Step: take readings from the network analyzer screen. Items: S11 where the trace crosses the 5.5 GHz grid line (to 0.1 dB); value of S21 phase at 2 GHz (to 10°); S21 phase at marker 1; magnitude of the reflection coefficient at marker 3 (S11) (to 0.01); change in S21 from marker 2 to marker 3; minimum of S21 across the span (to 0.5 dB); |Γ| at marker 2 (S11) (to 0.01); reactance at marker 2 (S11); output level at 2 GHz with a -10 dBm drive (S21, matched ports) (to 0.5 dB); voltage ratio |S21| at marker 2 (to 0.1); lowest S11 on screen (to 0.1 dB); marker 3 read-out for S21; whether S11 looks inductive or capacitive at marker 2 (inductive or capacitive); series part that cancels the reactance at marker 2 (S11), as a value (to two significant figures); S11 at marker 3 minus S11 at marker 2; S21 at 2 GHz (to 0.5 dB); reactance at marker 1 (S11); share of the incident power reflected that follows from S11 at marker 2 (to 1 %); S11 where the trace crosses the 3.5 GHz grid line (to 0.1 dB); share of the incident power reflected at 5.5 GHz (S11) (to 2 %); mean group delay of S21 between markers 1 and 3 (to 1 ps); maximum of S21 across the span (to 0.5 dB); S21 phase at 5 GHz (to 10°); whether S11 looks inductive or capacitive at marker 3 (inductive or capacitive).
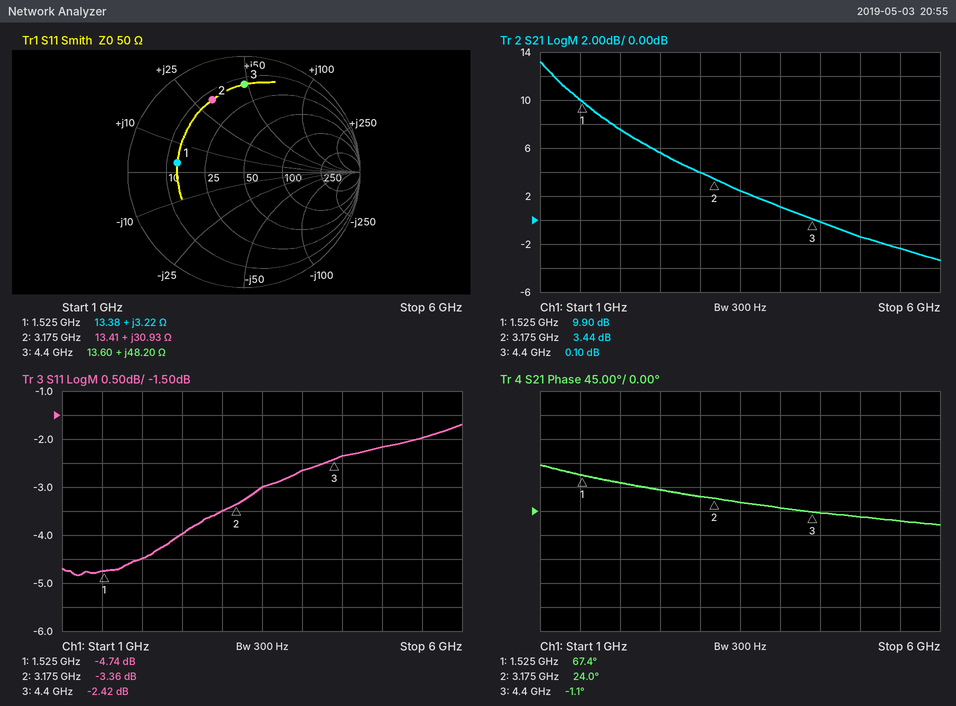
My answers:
-2.0 dB
50°
67.4°
0.76
-3.34 dB
-3.5 dB
0.68
+30.93 Ω
-2.5 dBm
1.5
-4.8 dB
0.10 dB
inductive
1.6 pF
0.94 dB
7.5 dB
+3.22 Ω
46 %
-3.0 dB
64 %
66 ps
13.0 dB
-10°
inductive
